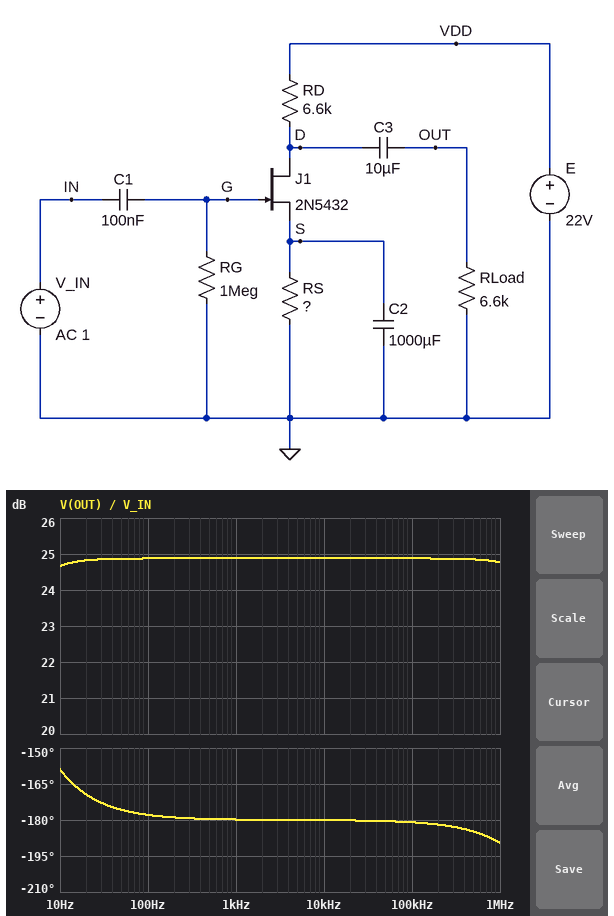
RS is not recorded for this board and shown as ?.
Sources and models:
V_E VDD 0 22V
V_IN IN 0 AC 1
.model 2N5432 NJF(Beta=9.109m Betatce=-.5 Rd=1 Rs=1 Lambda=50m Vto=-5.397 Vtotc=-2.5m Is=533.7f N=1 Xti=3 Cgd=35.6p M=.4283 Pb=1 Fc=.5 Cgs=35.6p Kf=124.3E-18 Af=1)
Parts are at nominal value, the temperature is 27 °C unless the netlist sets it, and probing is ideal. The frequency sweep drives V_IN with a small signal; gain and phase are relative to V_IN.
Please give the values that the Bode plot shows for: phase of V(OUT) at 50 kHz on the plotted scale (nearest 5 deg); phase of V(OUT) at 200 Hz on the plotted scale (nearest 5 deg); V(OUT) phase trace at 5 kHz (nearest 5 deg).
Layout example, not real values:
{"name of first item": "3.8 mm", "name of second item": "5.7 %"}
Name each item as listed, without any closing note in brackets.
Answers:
{"phase of V(OUT) at 50 kHz on the plotted scale": "-180 deg", "phase of V(OUT) at 200 Hz on the plotted scale": "-180 deg", "V(OUT) phase trace at 5 kHz": "-180 deg"}
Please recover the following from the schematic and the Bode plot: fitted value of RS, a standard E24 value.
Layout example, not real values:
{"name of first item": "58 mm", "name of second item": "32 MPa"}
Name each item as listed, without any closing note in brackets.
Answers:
{"fitted value of RS, a standard E24 value": "10 kΩ"}
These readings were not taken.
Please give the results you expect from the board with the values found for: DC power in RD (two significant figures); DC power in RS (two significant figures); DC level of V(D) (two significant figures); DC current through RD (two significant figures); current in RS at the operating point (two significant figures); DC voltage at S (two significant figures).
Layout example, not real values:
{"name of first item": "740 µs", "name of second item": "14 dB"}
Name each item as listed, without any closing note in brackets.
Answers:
{"DC power in RD": "1.8 mW", "DC power in RS": "2.7 mW", "DC level of V(D)": "19 V", "DC current through RD": "520 µA", "current in RS at the operating point": "520 µA", "DC voltage at S": "5.2 V"}
